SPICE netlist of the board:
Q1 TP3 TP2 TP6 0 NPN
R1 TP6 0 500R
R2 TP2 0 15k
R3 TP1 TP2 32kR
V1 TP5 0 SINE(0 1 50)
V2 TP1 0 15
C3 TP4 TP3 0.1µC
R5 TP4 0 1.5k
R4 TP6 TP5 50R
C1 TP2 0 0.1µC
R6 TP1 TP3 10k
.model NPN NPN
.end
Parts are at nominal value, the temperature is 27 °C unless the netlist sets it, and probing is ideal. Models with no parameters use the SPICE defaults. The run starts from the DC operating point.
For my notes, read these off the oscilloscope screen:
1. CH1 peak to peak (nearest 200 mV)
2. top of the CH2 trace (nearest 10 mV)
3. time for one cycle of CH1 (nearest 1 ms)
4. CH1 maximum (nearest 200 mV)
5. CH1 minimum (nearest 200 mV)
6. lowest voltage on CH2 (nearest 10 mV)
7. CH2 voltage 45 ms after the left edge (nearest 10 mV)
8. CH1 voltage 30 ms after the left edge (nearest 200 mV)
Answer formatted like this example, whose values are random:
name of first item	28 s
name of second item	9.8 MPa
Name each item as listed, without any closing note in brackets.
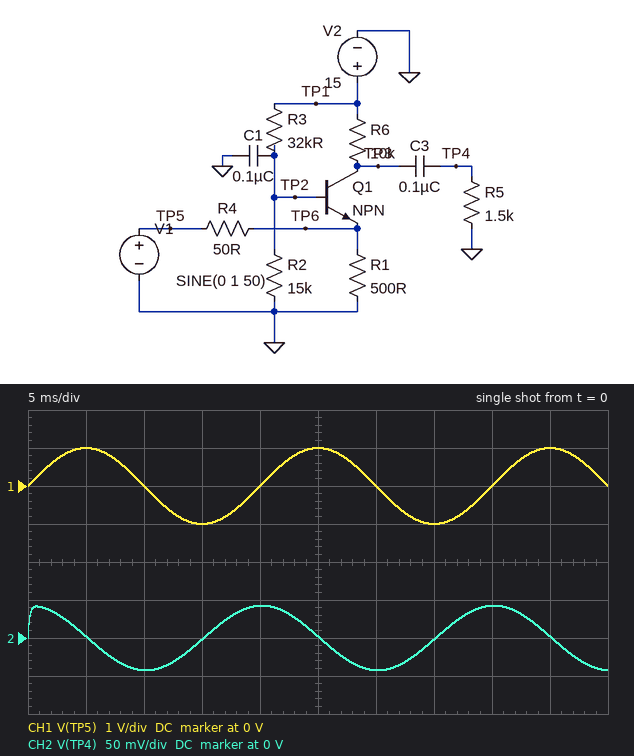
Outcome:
CH1 peak to peak	2.0 V
top of the CH2 trace	40 mV
time for one cycle of CH1	20 ms
CH1 maximum	1.0 V
CH1 minimum	-1.0 V
lowest voltage on CH2	-40 mV
CH2 voltage 45 ms after the left edge	0 V
CH1 voltage 30 ms after the left edge	0 V
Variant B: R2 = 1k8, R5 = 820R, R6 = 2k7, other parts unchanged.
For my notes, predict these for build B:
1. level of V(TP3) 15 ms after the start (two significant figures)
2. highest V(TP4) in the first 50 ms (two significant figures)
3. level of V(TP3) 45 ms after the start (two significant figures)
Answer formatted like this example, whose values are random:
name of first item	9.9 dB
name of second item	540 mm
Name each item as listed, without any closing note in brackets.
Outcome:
level of V(TP3) 15 ms after the start	-550 mV
highest V(TP4) in the first 50 ms	790 mV
level of V(TP3) 45 ms after the start	15 V
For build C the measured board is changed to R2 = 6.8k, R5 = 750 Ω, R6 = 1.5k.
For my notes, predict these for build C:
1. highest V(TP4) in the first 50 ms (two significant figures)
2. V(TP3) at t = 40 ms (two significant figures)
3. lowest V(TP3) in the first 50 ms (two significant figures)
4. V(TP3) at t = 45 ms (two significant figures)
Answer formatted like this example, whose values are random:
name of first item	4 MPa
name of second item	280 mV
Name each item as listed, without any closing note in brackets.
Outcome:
highest V(TP4) in the first 50 ms	47 mV
V(TP3) at t = 40 ms	560 mV
lowest V(TP3) in the first 50 ms	-330 mV
V(TP3) at t = 45 ms	2.0 V
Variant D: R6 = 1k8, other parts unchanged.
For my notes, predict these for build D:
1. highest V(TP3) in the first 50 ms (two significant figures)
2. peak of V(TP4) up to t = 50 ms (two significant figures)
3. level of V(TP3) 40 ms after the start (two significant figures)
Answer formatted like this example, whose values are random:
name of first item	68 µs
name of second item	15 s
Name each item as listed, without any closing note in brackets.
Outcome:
highest V(TP3) in the first 50 ms	1.4 V
peak of V(TP4) up to t = 50 ms	42 mV
level of V(TP3) 40 ms after the start	470 mV
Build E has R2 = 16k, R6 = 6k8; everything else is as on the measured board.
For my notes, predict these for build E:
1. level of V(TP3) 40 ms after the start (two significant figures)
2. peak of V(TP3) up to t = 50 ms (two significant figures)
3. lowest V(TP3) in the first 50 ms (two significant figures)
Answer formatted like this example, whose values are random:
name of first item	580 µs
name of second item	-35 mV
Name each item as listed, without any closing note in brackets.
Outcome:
level of V(TP3) 40 ms after the start	170 mV
peak of V(TP3) up to t = 50 ms	1.1 V
lowest V(TP3) in the first 50 ms	-730 mV
